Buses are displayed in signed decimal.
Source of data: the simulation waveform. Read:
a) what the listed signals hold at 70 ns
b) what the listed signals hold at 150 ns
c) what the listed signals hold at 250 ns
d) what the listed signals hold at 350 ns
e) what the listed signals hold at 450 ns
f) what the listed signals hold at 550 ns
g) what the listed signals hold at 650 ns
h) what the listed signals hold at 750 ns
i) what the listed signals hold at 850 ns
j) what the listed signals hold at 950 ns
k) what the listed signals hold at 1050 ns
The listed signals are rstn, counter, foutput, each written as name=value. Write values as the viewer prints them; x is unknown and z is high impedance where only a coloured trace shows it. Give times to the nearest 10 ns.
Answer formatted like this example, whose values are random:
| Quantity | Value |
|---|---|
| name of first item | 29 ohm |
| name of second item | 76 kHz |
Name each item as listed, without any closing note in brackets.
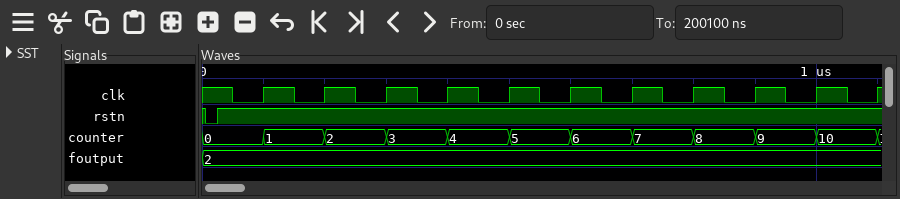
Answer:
| Quantity | Value |
|---|---|
| what the listed signals hold at 70 ns | rstn=1, counter=0, foutput=2 |
| what the listed signals hold at 150 ns | rstn=1, counter=1, foutput=2 |
| what the listed signals hold at 250 ns | rstn=1, counter=2, foutput=2 |
| what the listed signals hold at 350 ns | rstn=1, counter=3, foutput=2 |
| what the listed signals hold at 450 ns | rstn=1, counter=4, foutput=2 |
| what the listed signals hold at 550 ns | rstn=1, counter=5, foutput=2 |
| what the listed signals hold at 650 ns | rstn=1, counter=6, foutput=2 |
| what the listed signals hold at 750 ns | rstn=1, counter=7, foutput=2 |
| what the listed signals hold at 850 ns | rstn=1, counter=8, foutput=2 |
| what the listed signals hold at 950 ns | rstn=1, counter=9, foutput=2 |
| what the listed signals hold at 1050 ns | rstn=1, counter=10, foutput=2 |
